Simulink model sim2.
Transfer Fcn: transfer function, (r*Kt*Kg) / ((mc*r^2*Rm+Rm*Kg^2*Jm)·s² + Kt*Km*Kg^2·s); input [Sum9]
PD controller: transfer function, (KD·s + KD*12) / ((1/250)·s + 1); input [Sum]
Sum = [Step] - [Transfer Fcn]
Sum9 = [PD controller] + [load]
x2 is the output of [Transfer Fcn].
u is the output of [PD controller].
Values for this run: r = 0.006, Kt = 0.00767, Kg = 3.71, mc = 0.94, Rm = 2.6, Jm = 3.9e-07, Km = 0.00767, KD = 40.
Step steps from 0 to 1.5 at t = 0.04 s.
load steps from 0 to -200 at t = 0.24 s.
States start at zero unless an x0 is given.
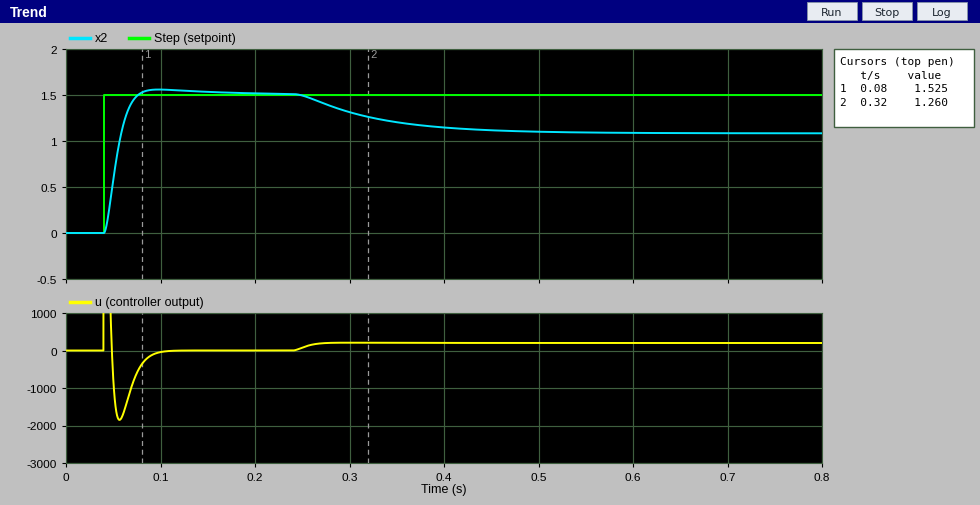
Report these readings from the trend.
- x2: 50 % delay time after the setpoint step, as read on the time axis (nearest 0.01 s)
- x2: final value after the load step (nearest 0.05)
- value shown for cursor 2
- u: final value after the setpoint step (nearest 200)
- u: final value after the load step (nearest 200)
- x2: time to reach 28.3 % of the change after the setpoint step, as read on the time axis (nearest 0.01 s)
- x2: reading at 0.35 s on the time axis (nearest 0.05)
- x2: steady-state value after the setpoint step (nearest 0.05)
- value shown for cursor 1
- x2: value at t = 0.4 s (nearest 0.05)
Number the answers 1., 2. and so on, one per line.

1. 0.05 s
2. 1.10
3. 1.260
4. 0
5. 200
6. 0.05 s
7. 1.20
8. 1.50
9. 1.525
10. 1.15
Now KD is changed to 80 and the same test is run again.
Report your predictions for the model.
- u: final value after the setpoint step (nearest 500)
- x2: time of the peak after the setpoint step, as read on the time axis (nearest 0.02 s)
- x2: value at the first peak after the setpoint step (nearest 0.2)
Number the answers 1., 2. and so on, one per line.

1. 0
2. 0.06 s
3. 1.6
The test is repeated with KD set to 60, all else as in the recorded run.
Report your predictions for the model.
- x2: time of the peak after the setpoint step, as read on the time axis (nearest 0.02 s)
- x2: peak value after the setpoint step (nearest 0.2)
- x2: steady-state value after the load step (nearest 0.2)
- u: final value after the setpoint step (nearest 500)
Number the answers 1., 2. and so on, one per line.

1. 0.08 s
2. 1.6
3. 1.2
4. 0
